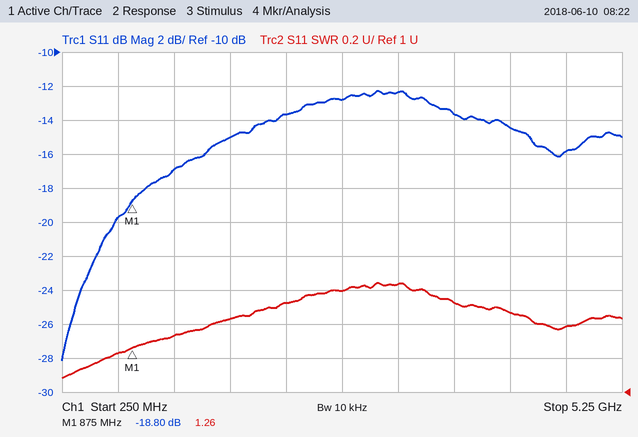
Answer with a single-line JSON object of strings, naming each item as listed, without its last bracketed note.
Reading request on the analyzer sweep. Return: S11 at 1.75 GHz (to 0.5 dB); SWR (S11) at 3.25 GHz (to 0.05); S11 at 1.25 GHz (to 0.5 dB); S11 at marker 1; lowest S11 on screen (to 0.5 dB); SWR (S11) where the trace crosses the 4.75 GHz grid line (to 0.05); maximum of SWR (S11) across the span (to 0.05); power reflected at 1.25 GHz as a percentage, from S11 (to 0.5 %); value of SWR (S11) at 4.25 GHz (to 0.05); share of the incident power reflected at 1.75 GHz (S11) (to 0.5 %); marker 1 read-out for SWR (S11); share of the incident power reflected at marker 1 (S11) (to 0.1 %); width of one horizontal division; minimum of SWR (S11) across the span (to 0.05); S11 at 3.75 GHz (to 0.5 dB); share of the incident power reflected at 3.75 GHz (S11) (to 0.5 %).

{"S11 at 1.75 GHz": "-15.0 dB", "SWR (S11) at 3.25 GHz": "1.65", "S11 at 1.25 GHz": "-17.0 dB", "S11 at marker 1": "-18.80 dB", "lowest S11 on screen": "-28.0 dB", "SWR (S11) where the trace crosses the 4.75 GHz grid line": "1.40", "maximum of SWR (S11) across the span": "1.65", "power reflected at 1.25 GHz as a percentage, from S11": "2.0 %", "value of SWR (S11) at 4.25 GHz": "1.45", "share of the incident power reflected at 1.75 GHz (S11)": "3.0 %", "marker 1 read-out for SWR": "1.26", "share of the incident power reflected at marker 1 (S11)": "1.3 %", "width of one horizontal division": "500 MHz", "minimum of SWR (S11) across the span": "1.10", "S11 at 3.75 GHz": "-13.5 dB", "share of the incident power reflected at 3.75 GHz (S11)": "4.5 %"}
